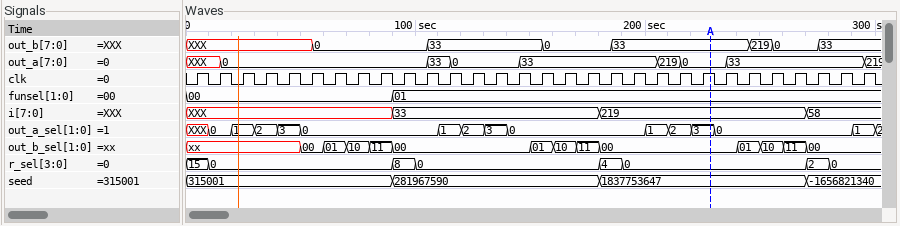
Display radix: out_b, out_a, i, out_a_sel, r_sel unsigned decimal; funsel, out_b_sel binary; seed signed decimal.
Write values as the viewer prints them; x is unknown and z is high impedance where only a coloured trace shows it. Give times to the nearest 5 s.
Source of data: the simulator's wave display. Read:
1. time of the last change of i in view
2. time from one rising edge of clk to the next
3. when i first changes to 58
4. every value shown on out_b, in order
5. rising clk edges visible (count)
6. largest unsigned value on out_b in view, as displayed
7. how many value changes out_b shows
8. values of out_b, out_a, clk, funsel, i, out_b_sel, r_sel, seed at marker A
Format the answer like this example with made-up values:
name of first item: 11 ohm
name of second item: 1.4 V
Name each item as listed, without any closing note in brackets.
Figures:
time of the last change of i in view: 270 s
time from one rising edge of clk to the next: 10 s
when i first changes to 58: 270 s
every value shown on out_b, in order: XXX, 0, 33, 0, 33, 219, 0, 33
rising clk edges visible: 30
largest unsigned value on out_b in view, as displayed: 219
how many value changes out_b shows: 7
values of out_b, out_a, clk, funsel, i, out_b_sel, r_sel, seed at marker A: out_b=33, out_a=0, clk=1, funsel=01, i=219, out_b_sel=00, r_sel=0, seed=1837753647
